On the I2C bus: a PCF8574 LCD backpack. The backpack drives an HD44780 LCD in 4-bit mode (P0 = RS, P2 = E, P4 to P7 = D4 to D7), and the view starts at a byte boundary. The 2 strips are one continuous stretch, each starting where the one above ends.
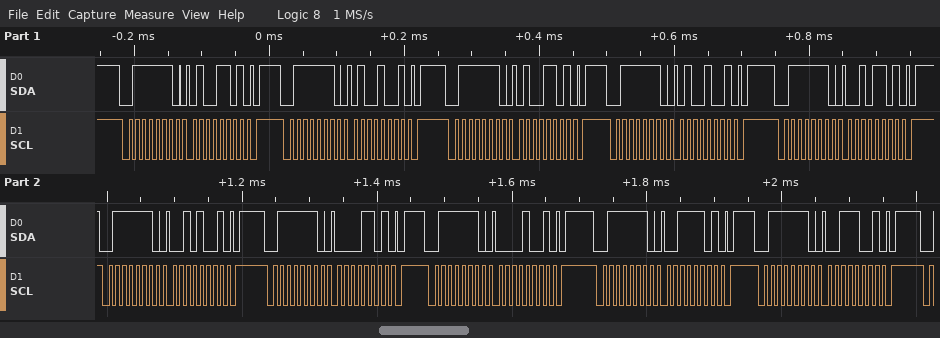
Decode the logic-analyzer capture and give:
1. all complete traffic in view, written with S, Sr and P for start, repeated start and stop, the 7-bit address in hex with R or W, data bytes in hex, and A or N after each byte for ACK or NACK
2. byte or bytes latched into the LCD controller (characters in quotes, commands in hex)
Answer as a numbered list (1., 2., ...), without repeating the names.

1. S 3FW A 4D A P S 3FW A 49 A P S 3FW A 4D A P S 3FW A 49 A P S 3FW A 2D A P S 3FW A 29 A P S 3FW A 0D A P S 3FW A 09 A P S 3FW A 3D A P S 3FW A 39 A P
2. 'D' ' '
